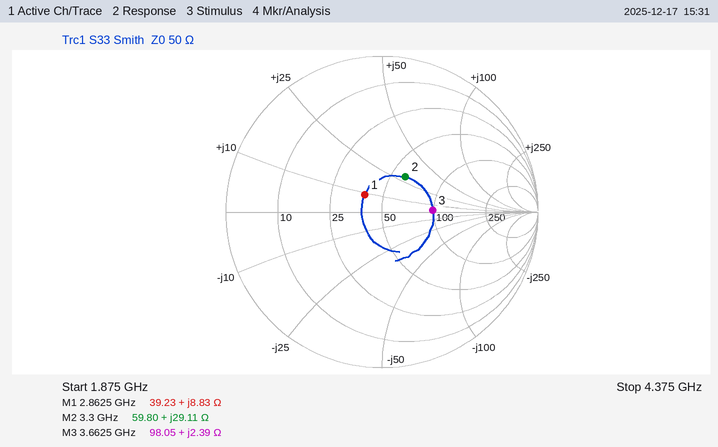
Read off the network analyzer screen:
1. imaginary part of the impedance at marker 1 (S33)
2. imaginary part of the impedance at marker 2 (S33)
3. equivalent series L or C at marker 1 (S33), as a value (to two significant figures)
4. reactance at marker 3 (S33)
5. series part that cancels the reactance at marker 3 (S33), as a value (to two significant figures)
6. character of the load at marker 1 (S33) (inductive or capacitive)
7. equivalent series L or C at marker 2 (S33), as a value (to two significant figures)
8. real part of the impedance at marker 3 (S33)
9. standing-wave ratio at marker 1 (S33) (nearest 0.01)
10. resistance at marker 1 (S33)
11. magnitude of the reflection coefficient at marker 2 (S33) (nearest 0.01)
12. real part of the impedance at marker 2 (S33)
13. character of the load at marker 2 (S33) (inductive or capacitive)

+8.83 Ω
+29.11 Ω
490 pH
+2.39 Ω
18 pF
inductive
1.4 nH
98.05 Ω
1.37
39.23 Ω
0.27
59.80 Ω
inductive
